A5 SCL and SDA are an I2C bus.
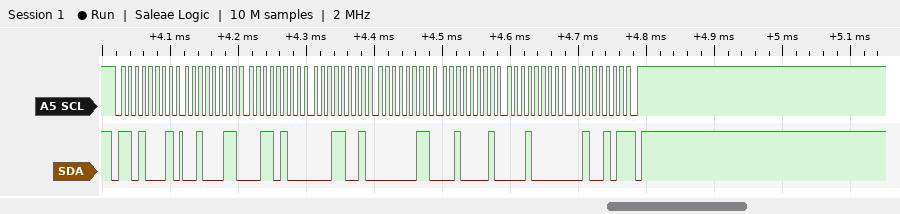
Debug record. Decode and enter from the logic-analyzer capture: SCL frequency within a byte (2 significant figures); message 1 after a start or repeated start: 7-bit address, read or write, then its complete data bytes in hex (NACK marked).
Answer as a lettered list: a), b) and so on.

a) 100 kHz
b) 0x68 read: 23 34 19 03 21 10 25 NACK
